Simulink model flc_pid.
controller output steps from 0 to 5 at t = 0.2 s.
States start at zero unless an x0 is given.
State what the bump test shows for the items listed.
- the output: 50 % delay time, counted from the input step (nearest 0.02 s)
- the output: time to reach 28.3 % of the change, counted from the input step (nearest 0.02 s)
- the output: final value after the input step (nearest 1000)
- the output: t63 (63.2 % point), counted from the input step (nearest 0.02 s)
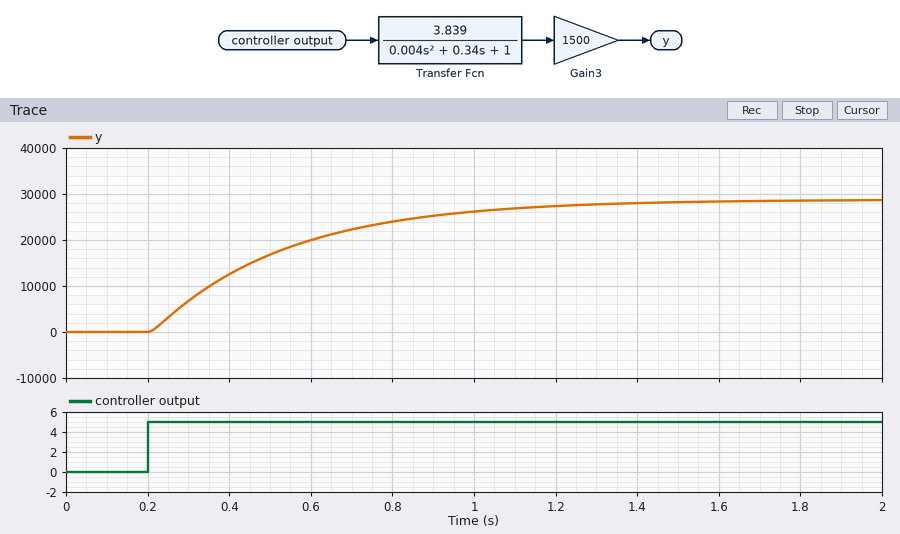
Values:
0.24 s
0.12 s
29000
0.34 s
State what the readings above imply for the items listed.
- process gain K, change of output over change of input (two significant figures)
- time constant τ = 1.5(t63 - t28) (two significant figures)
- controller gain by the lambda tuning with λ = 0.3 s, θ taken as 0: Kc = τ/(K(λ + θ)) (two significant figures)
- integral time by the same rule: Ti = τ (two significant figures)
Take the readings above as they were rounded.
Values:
5800
0.33 s
0.00019
0.33 s
